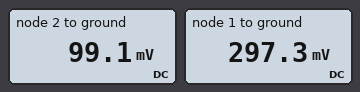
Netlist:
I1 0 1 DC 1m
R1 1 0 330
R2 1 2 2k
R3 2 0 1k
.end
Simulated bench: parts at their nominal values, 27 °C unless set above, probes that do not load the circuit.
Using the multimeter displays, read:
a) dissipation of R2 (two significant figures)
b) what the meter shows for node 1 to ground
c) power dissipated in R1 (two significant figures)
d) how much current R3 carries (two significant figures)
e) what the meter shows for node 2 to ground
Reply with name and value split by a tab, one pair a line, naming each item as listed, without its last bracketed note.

dissipation of R2	20 µW
what the meter shows for node 1 to ground	297.3 mV
power dissipated in R1	270 µW
how much current R3 carries	99 µA
what the meter shows for node 2 to ground	99.1 mV
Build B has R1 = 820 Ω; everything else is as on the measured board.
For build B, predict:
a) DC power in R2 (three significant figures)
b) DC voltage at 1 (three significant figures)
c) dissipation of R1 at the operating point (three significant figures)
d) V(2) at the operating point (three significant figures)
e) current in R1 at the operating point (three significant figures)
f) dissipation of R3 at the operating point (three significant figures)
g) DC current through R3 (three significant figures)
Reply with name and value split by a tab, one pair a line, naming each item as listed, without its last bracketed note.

DC power in R2	92.2 µW
DC voltage at 1	644 mV
dissipation of R1 at the operating point	506 µW
V(2) at the operating point	215 mV
current in R1 at the operating point	785 µA
dissipation of R3 at the operating point	46.1 µW
DC current through R3	215 µA
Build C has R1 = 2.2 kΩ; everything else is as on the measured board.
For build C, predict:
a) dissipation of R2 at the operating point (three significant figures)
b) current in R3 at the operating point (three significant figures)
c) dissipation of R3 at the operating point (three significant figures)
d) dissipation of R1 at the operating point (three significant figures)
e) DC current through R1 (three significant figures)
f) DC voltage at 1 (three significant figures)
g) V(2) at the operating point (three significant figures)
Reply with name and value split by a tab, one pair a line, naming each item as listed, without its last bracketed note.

dissipation of R2 at the operating point	358 µW
current in R3 at the operating point	423 µA
dissipation of R3 at the operating point	179 µW
dissipation of R1 at the operating point	732 µW
DC current through R1	577 µA
DC voltage at 1	1.27 V
V(2) at the operating point	423 mV
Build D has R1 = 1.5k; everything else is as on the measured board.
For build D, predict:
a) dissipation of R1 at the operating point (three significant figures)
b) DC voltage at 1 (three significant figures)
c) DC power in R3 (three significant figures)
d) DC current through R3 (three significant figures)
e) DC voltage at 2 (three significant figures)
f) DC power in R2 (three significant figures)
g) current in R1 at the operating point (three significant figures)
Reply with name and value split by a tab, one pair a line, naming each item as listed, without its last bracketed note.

dissipation of R1 at the operating point	667 µW
DC voltage at 1	1.00 V
DC power in R3	111 µW
DC current through R3	333 µA
DC voltage at 2	333 mV
DC power in R2	222 µW
current in R1 at the operating point	667 µA
